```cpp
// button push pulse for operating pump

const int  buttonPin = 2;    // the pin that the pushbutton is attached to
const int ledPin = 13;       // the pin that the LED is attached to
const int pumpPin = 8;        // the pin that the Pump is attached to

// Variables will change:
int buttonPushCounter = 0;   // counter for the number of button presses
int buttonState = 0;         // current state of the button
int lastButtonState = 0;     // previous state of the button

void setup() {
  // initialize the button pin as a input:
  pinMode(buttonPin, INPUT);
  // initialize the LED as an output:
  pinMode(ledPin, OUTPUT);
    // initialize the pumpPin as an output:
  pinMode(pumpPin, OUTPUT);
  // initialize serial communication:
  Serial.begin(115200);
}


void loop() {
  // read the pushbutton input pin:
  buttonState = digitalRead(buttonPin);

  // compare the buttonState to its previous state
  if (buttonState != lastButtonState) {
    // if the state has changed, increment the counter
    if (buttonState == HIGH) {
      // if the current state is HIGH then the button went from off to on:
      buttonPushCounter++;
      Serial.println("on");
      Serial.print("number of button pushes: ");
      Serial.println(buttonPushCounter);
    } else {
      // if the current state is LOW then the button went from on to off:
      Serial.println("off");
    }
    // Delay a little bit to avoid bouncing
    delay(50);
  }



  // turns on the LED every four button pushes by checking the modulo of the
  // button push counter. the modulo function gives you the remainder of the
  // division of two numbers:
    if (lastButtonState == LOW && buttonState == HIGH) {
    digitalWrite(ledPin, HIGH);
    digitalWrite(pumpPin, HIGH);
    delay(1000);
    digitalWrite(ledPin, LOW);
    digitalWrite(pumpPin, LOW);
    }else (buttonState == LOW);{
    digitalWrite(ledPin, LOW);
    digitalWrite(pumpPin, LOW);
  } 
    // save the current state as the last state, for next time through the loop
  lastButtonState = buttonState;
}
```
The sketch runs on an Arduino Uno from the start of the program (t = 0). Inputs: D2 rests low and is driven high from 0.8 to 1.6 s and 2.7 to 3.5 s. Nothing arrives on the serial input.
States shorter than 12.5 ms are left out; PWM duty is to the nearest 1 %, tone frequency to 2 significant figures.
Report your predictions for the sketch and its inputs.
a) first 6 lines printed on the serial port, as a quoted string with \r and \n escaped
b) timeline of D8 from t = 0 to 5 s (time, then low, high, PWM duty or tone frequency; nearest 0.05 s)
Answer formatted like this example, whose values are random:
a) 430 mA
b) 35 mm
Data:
a) "on\r\nnumber of button pushes: 1\r\noff\r\non\r\nnumber of button pushes: 2\r\noff\r\n"
b) 0 s low; 0.85 s high; 1.85 s low; 2.75 s high; 3.75 s low
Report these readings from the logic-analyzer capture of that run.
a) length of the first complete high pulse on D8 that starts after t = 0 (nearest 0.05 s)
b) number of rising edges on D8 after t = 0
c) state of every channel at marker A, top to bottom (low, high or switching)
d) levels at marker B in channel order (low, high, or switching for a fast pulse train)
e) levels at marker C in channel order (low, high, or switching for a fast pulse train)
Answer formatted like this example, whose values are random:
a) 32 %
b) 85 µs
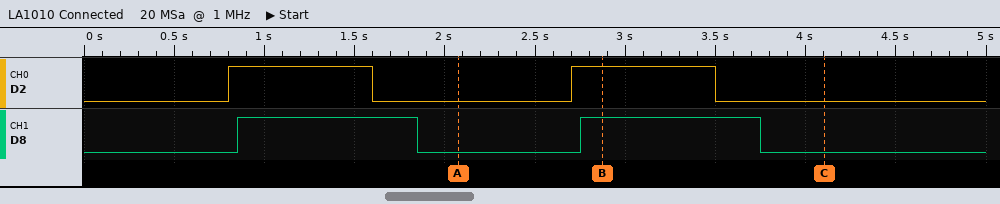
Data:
a) 1.00 s
b) 2
c) D2 low, D8 low
d) D2 high, D8 high
e) D2 low, D8 low
